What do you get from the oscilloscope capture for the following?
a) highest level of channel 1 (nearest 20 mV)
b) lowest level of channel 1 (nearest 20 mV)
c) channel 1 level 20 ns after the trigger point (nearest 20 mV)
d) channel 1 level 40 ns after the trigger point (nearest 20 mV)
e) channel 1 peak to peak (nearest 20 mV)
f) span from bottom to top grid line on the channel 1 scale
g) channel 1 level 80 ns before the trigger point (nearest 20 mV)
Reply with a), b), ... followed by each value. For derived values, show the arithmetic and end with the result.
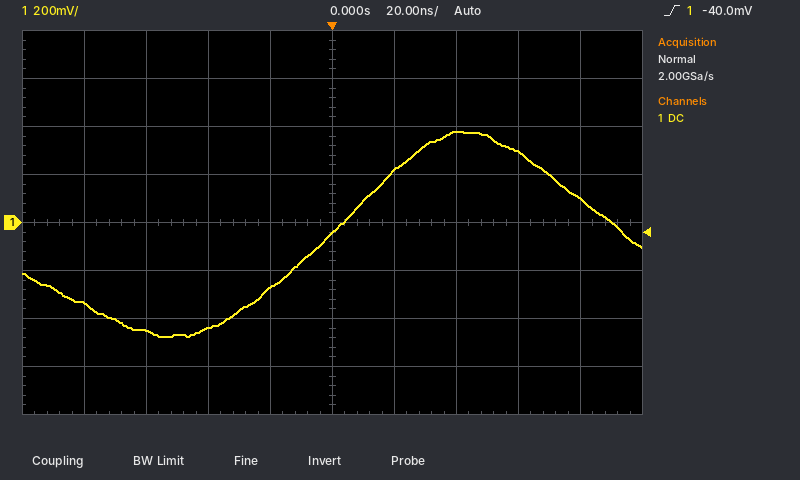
a) 380 mV
b) -480 mV
c) 220 mV
d) 380 mV
e) 380 mV − (-480 mV) = 860 mV
f) 1.6 V
g) -340 mV
